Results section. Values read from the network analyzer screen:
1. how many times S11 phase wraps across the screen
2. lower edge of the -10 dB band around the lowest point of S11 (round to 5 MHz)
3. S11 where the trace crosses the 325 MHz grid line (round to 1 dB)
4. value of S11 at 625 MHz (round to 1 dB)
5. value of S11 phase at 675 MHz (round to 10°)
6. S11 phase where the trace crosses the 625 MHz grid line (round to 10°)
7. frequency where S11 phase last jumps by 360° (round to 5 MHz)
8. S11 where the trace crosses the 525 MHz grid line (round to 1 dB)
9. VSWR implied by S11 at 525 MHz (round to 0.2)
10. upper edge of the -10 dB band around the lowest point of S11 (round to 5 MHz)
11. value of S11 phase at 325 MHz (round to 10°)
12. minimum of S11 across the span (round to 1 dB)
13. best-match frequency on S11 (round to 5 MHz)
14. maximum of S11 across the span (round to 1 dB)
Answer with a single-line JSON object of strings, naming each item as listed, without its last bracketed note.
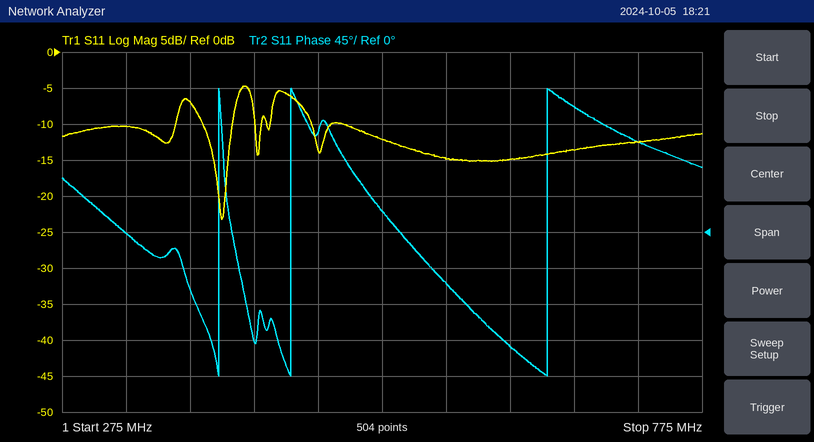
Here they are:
{"how many times S11 phase wraps across the screen": "3", "lower edge of the -10 dB band around the lowest point of S11": "385 MHz", "S11 where the trace crosses the 325 MHz grid line": "-10 dB", "value of S11 at 625 MHz": "-15 dB", "value of S11 phase at 675 MHz": "160°", "S11 phase where the trace crosses the 625 MHz grid line": "-140°", "frequency where S11 phase last jumps by 360°": "655 MHz", "S11 where the trace crosses the 525 MHz grid line": "-12 dB", "VSWR implied by S11 at 525 MHz": "1.6", "upper edge of the -10 dB band around the lowest point of S11": "410 MHz", "value of S11 phase at 325 MHz": "0°", "minimum of S11 across the span": "-23 dB", "best-match frequency on S11": "400 MHz", "maximum of S11 across the span": "-5 dB"}
